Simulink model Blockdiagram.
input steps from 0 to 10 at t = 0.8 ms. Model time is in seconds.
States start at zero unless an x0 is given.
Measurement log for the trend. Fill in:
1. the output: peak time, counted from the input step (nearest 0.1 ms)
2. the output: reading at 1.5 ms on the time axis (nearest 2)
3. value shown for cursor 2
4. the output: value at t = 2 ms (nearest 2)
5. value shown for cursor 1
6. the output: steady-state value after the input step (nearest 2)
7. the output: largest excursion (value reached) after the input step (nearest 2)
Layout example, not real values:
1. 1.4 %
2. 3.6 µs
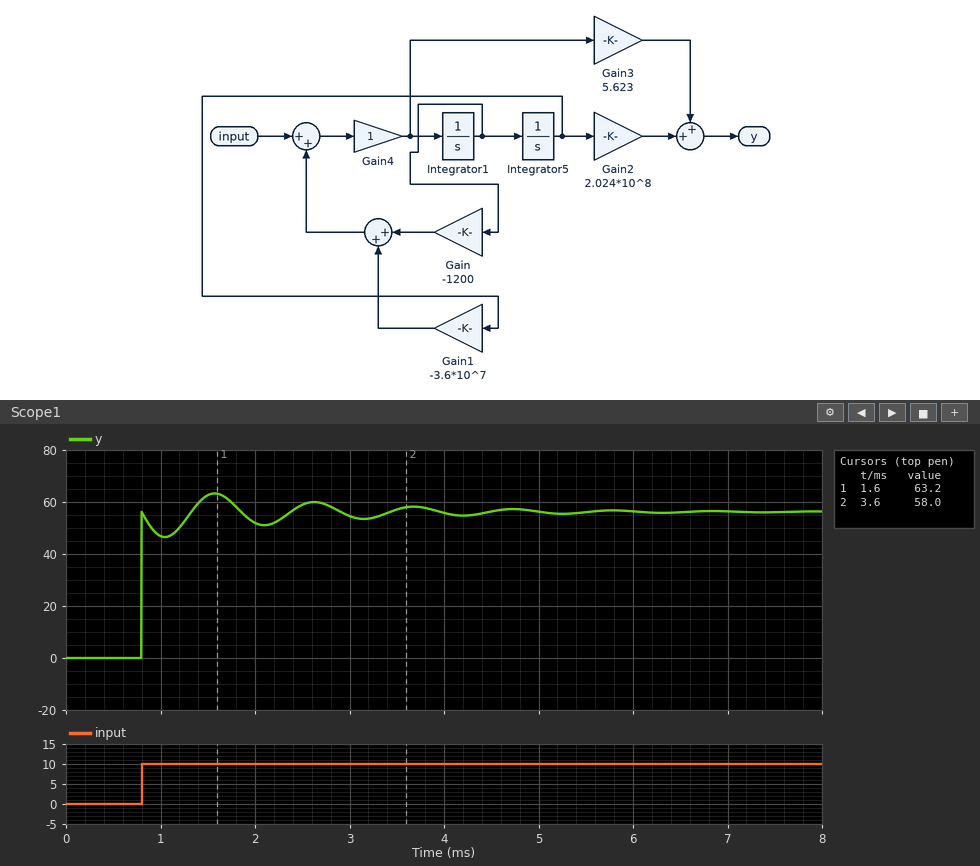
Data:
1. 0.8 ms
2. 62
3. 58.0
4. 52
5. 63.2
6. 56
7. 64
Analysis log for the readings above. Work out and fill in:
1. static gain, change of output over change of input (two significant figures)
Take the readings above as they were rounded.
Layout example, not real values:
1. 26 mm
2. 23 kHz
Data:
1. 5.6
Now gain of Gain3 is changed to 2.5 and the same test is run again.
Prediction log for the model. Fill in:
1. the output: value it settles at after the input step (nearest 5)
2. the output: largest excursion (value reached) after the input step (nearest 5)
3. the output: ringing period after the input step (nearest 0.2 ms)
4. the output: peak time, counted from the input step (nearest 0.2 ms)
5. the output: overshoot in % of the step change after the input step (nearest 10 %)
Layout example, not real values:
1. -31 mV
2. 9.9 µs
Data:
1. 55
2. 80
3. 1.0 ms
4. 0.6 ms
5. 40 %
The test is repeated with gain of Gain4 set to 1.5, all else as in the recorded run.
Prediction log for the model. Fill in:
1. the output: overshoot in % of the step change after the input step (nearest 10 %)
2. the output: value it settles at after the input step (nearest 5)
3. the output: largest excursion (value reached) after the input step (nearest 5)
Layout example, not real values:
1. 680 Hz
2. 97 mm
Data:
1. 50 %
2. 55
3. 85
